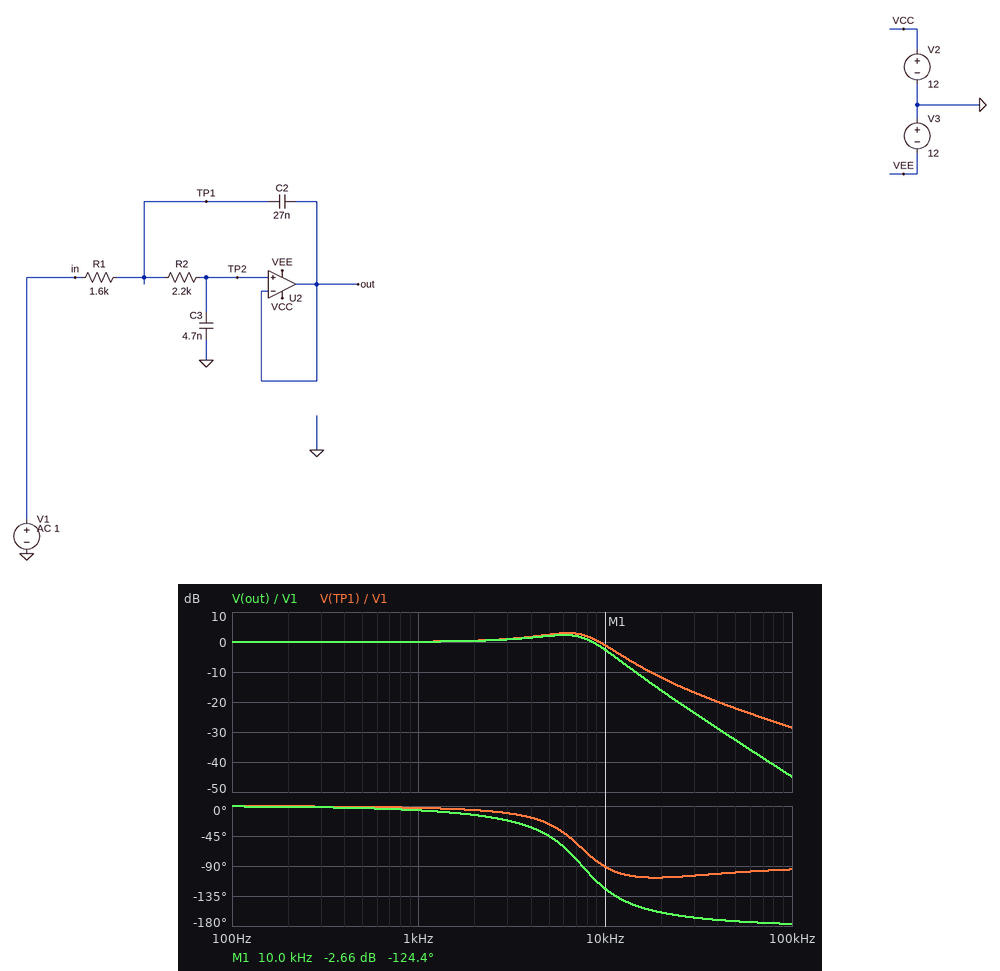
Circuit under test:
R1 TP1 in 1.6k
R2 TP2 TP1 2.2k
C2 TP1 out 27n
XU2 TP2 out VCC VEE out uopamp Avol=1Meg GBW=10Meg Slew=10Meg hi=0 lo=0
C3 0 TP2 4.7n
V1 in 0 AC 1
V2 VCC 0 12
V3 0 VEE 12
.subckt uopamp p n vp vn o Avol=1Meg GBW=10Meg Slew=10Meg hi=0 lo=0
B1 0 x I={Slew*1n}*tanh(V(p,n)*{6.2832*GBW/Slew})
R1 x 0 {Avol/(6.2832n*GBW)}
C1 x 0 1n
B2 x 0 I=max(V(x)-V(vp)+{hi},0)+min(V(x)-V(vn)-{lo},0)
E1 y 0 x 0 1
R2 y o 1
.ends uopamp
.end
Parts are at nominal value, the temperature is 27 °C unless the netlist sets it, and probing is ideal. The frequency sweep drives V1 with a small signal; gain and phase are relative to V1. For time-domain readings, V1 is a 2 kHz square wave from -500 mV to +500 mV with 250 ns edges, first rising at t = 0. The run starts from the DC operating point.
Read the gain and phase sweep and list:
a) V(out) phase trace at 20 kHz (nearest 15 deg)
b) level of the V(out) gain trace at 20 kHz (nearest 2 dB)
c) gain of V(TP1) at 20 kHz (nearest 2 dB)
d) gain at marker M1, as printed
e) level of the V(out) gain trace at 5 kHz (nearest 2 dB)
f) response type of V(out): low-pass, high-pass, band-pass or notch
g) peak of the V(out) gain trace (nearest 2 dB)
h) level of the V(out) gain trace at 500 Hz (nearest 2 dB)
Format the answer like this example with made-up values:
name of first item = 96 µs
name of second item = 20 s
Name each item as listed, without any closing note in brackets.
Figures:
V(out) phase trace at 20 kHz = -165 deg
level of the V(out) gain trace at 20 kHz = -16 dB
gain of V(TP1) at 20 kHz = -12 dB
gain at marker M1, as printed = -2.66 dB
level of the V(out) gain trace at 5 kHz = 2 dB
response type of V(out): low-pass, high-pass, band-pass or notch = low-pass
peak of the V(out) gain trace = 2 dB
level of the V(out) gain trace at 500 Hz = 0 dB
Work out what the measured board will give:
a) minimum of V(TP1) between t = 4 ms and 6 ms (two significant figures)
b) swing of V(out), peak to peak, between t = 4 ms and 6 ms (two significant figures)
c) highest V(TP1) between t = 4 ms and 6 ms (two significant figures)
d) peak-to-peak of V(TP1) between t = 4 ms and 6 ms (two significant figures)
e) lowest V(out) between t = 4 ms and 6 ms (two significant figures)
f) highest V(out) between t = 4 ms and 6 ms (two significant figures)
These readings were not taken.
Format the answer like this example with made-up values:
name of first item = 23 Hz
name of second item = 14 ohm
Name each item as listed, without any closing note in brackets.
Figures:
minimum of V(TP1) between t = 4 ms and 6 ms = -770 mV
swing of V(out), peak to peak, between t = 4 ms and 6 ms = 1.5 V
highest V(TP1) between t = 4 ms and 6 ms = 770 mV
peak-to-peak of V(TP1) between t = 4 ms and 6 ms = 1.5 V
lowest V(out) between t = 4 ms and 6 ms = -730 mV
highest V(out) between t = 4 ms and 6 ms = 730 mV
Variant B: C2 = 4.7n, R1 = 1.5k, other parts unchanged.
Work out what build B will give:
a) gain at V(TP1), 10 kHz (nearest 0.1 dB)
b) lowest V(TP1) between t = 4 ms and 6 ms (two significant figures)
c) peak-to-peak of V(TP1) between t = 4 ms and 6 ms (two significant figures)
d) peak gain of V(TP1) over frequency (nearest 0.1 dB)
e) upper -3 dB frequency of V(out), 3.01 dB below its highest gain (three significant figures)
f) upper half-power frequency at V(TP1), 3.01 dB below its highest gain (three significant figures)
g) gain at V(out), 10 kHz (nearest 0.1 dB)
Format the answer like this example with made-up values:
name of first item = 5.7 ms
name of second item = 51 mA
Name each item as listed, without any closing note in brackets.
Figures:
gain at V(TP1), 10 kHz = -0.8 dB
lowest V(TP1) between t = 4 ms and 6 ms = -500 mV
peak-to-peak of V(TP1) between t = 4 ms and 6 ms = 1.0 V
peak gain of V(TP1) over frequency = 0 dB
upper -3 dB frequency of V(out), 3.01 dB below its highest gain = 11.7 kHz
upper half-power frequency at V(TP1), 3.01 dB below its highest gain = 22.6 kHz
gain at V(out), 10 kHz = -2.3 dB
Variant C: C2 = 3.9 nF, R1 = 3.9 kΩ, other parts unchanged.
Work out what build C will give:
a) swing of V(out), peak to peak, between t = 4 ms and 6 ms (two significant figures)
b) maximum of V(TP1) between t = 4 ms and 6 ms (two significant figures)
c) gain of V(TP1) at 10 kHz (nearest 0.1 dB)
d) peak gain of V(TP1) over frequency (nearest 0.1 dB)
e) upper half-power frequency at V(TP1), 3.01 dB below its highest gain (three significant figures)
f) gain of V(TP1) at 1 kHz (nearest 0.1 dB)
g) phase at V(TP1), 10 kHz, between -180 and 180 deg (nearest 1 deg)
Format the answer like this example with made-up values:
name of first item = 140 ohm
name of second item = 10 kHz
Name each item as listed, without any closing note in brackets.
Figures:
swing of V(out), peak to peak, between t = 4 ms and 6 ms = 1.0 V
maximum of V(TP1) between t = 4 ms and 6 ms = 500 mV
gain of V(TP1) at 10 kHz = -3.8 dB
peak gain of V(TP1) over frequency = 0 dB
upper half-power frequency at V(TP1), 3.01 dB below its highest gain = 8.37 kHz
gain of V(TP1) at 1 kHz = -0.1 dB
phase at V(TP1), 10 kHz, between -180 and 180 deg = -45 deg
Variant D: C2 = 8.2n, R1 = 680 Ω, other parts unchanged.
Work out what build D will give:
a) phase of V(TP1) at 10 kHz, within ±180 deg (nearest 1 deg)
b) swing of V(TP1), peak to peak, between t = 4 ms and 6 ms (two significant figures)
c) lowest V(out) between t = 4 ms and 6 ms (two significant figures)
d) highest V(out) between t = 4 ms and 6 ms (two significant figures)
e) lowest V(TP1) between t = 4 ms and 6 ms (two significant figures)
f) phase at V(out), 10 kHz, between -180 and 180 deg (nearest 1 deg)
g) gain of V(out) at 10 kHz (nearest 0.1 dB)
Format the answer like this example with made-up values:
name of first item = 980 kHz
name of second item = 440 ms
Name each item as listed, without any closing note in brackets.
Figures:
phase of V(TP1) at 10 kHz, within ±180 deg = -15 deg
swing of V(TP1), peak to peak, between t = 4 ms and 6 ms = 1.1 V
lowest V(out) between t = 4 ms and 6 ms = -500 mV
highest V(out) between t = 4 ms and 6 ms = 500 mV
lowest V(TP1) between t = 4 ms and 6 ms = -560 mV
phase at V(out), 10 kHz, between -180 and 180 deg = -48 deg
gain of V(out) at 10 kHz = -1.2 dB
